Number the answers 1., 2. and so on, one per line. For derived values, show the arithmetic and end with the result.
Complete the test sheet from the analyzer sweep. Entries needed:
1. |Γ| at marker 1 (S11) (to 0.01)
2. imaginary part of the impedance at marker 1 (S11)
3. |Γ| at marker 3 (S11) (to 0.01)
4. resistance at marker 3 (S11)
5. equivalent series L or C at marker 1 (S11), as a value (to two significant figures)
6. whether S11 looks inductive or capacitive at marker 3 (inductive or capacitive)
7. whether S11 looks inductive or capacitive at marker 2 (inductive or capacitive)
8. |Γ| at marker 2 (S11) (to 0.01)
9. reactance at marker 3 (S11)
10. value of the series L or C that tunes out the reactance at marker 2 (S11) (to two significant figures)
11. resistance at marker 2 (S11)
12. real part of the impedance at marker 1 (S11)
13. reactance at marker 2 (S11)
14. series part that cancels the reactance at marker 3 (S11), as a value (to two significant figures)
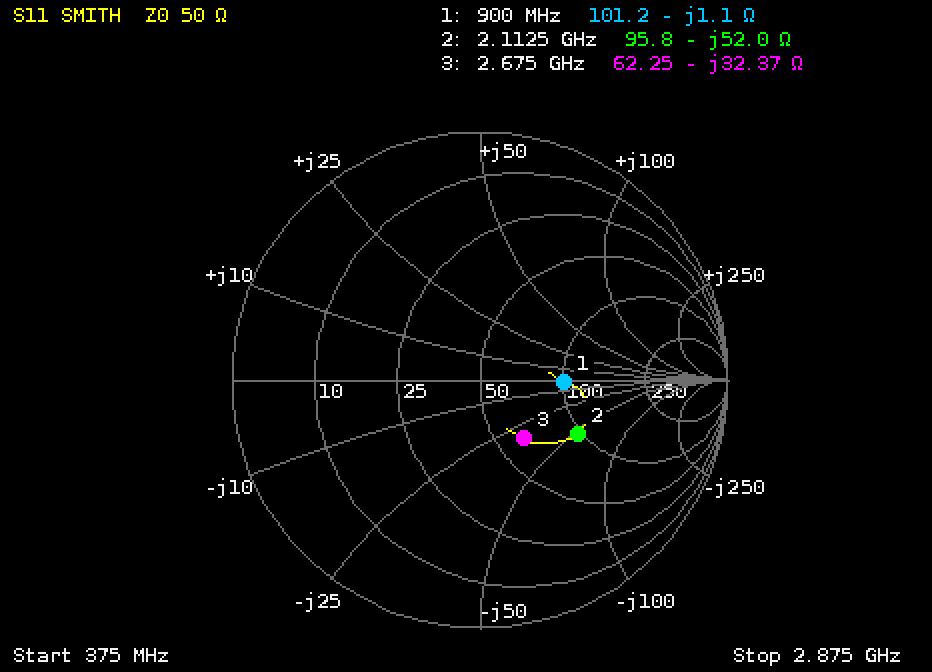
1. 0.34
2. -1.1 Ω
3. 0.30
4. 62.25 Ω
5. C = 1/(2π × 900 MHz × 1.1 Ω) ≈ 161 pF, so 160 pF to two significant figures
6. capacitive
7. capacitive
8. 0.45
9. -32.37 Ω
10. L = 52 Ω/(2π × 2.1125 GHz) ≈ 3.9 nH
11. 95.8 Ω
12. 101.2 Ω
13. -52.0 Ω
14. L = 32.37 Ω/(2π × 2.675 GHz) ≈ 1.9 nH
